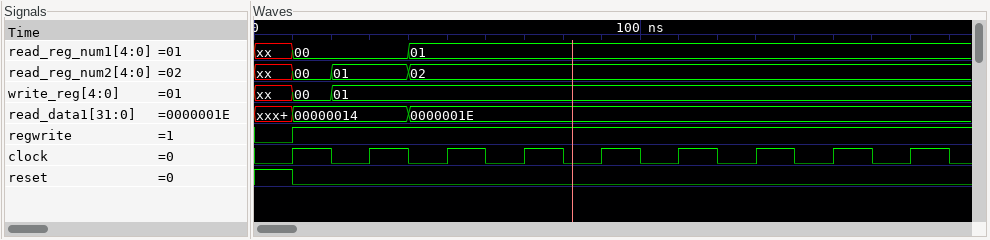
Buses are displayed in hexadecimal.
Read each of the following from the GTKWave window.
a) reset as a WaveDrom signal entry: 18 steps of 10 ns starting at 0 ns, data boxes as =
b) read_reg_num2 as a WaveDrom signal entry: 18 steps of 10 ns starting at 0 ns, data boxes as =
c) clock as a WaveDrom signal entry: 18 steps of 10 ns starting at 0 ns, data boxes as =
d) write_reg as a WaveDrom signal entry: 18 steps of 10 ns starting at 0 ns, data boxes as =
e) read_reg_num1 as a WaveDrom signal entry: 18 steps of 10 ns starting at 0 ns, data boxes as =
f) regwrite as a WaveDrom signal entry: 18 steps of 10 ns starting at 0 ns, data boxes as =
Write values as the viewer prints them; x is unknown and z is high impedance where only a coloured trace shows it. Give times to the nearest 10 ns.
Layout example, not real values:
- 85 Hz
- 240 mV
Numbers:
- {name: 'reset', wave: '10................'}
- {name: 'read_reg_num2', wave: 'x==.=.............', data: '00 01 02'}
- {name: 'clock', wave: '010101010101010101'}
- {name: 'write_reg', wave: 'x==...............', data: '00 01'}
- {name: 'read_reg_num1', wave: 'x=..=.............', data: '00 01'}
- {name: 'regwrite', wave: '01................'}
